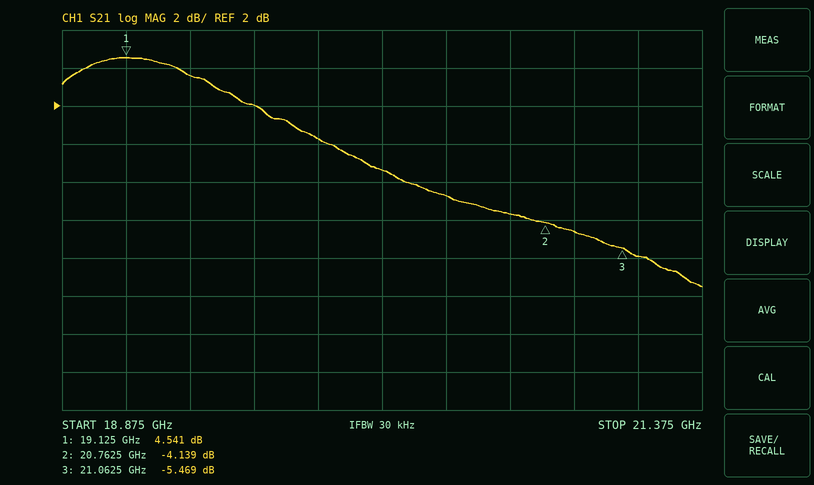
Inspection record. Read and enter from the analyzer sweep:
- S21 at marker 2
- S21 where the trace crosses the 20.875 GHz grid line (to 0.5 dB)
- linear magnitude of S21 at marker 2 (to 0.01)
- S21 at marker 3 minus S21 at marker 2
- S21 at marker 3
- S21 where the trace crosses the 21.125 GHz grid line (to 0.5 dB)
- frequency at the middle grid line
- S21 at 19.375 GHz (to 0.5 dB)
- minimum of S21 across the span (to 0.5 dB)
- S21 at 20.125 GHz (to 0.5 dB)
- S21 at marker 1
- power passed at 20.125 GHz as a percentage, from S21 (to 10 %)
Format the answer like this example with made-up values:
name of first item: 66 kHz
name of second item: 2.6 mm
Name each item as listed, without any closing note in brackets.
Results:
S21 at marker 2: -4.139 dB
S21 where the trace crosses the 20.875 GHz grid line: -4.5 dB
linear magnitude of S21 at marker 2: 0.62
S21 at marker 3 minus S21 at marker 2: -1.330 dB
S21 at marker 3: -5.469 dB
S21 where the trace crosses the 21.125 GHz grid line: -6.0 dB
frequency at the middle grid line: 20.125 GHz
S21 at 19.375 GHz: 3.5 dB
minimum of S21 across the span: -7.5 dB
S21 at 20.125 GHz: -1.5 dB
S21 at marker 1: 4.541 dB
power passed at 20.125 GHz as a percentage, from S21: 70 %
